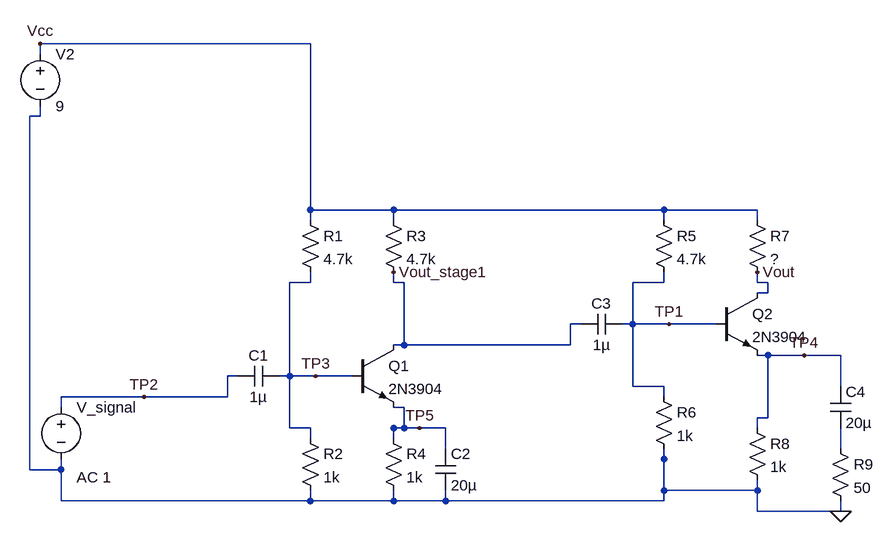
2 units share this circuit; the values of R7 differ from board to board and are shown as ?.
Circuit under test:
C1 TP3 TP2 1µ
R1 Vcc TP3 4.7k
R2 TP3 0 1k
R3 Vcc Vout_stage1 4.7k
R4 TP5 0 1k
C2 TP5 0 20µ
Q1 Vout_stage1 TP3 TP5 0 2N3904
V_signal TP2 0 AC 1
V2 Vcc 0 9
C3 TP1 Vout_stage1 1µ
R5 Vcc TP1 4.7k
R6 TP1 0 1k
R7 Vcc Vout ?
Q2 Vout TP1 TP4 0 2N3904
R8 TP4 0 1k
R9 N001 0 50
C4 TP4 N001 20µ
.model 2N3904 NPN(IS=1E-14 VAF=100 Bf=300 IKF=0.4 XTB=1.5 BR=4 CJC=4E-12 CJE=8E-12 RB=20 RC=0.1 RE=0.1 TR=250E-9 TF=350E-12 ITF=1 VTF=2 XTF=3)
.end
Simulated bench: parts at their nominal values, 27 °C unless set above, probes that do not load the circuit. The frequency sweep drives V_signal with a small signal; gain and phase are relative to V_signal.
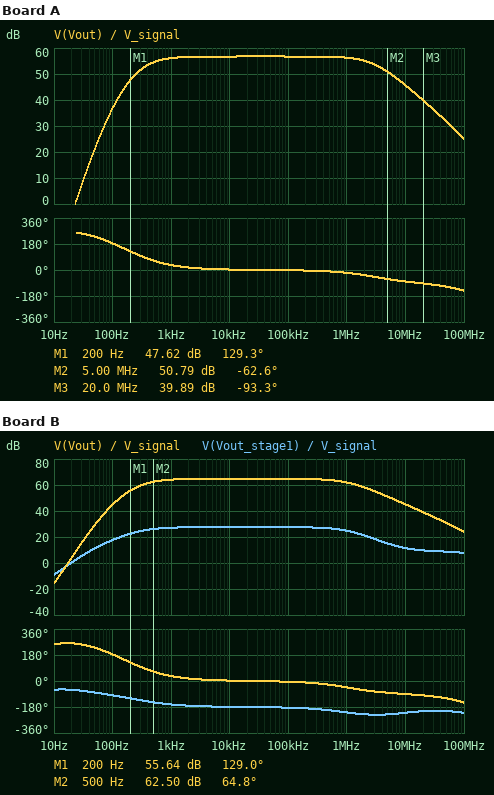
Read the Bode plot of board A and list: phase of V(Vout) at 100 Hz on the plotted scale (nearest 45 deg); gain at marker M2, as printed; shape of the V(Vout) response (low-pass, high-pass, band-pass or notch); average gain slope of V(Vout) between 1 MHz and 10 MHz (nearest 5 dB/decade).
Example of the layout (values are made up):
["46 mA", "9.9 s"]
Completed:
["180 deg", "50.79 dB", "band-pass", "-10 dB/decade"]
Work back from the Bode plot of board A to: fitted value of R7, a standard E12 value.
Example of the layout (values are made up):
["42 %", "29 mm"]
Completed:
["2.2 kΩ"]
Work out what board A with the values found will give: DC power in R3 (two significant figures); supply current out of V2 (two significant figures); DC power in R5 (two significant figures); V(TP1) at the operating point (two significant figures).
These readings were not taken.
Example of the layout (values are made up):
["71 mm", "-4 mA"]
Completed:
["4.0 mW", "5.0 mA", "12 mW", "1.6 V"]
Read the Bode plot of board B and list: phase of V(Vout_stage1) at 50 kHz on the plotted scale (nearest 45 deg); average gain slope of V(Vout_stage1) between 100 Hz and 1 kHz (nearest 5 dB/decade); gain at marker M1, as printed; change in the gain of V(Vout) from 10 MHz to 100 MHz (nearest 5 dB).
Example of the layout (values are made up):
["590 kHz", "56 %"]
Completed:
["-180 deg", "10 dB/decade", "55.64 dB", "-20 dB"]
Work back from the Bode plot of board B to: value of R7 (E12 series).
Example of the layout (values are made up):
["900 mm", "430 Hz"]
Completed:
["5.6 kΩ"]
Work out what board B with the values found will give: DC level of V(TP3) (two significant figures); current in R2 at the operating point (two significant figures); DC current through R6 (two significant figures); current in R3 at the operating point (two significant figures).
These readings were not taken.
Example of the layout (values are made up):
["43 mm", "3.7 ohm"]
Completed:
["1.6 V", "1.6 mA", "1.6 mA", "920 µA"]
